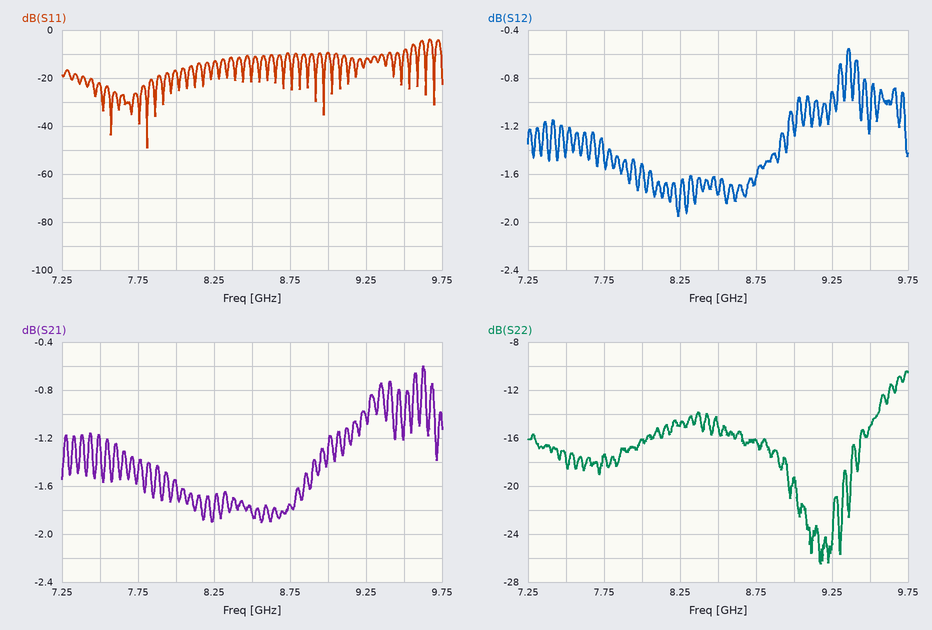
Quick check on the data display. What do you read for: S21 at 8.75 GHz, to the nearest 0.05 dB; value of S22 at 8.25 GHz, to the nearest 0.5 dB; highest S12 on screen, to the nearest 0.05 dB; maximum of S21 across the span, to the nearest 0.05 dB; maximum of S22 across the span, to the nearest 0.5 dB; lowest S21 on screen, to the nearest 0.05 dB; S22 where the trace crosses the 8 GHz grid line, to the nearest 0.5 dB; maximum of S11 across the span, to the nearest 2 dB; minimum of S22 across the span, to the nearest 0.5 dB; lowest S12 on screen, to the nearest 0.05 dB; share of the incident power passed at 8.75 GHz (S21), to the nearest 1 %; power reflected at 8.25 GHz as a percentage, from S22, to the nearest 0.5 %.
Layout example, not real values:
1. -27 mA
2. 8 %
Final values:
1. -1.75 dB
2. -15.0 dB
3. -0.55 dB
4. -0.60 dB
5. -10.5 dB
6. -1.90 dB
7. -16.0 dB
8. -4 dB
9. -26.5 dB
10. -1.95 dB
11. 67 %
12. 3.0 %
